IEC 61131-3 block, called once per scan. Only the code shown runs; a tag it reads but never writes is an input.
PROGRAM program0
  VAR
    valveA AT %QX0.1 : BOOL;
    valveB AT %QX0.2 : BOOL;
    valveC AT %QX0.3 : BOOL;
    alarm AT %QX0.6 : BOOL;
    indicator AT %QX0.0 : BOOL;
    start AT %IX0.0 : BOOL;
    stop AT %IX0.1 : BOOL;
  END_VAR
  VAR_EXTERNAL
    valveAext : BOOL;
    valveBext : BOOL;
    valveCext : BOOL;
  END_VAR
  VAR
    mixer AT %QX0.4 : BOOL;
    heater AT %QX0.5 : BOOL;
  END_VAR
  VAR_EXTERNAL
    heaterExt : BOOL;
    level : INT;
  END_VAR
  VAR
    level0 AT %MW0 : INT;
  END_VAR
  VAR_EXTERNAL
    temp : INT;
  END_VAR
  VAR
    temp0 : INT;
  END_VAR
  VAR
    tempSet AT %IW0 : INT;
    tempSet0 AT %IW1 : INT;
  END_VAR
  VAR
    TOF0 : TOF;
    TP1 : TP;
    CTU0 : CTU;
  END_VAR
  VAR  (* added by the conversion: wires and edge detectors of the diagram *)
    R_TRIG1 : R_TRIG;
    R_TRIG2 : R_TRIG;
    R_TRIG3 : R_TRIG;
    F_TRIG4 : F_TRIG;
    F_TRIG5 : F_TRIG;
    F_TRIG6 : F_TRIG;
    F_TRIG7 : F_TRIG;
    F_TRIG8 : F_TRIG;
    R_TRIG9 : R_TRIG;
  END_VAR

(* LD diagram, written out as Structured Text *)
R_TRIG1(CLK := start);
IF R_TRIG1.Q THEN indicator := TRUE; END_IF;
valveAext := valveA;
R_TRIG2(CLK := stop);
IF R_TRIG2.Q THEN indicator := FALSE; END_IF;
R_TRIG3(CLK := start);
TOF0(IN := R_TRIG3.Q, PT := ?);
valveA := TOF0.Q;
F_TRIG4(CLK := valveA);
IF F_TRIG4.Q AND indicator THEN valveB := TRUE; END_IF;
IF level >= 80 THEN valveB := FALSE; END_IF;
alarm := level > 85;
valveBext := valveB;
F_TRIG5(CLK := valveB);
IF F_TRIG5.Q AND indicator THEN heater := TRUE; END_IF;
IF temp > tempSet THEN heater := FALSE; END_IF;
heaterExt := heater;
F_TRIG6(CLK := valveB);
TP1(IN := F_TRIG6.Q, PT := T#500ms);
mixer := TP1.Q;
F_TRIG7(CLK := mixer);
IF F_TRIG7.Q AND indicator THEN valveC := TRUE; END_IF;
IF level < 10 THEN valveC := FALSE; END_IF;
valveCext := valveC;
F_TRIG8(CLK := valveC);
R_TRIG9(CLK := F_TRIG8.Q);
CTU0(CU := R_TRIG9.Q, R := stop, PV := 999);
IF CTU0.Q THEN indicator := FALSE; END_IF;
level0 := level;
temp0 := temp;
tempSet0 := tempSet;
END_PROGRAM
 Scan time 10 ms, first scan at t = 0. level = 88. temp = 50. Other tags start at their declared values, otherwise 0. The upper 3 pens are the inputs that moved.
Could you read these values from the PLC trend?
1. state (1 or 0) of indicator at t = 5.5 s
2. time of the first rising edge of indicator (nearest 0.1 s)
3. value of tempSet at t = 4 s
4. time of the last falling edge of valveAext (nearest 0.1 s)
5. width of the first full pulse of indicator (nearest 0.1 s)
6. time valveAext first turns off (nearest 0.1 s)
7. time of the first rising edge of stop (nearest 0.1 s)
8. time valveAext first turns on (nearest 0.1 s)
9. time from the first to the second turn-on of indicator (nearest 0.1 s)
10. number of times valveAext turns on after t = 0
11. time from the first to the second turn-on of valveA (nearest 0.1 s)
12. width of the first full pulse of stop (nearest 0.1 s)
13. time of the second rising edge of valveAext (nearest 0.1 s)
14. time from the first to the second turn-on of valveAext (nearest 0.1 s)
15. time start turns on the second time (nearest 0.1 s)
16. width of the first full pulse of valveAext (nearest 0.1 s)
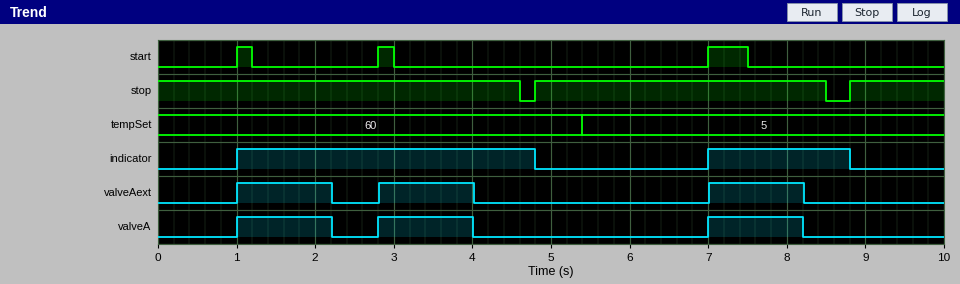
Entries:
0
1.0 s
60
8.2 s
3.8 s
2.2 s
4.8 s
1.0 s
6.0 s
3
1.8 s
3.7 s
2.8 s
1.8 s
2.8 s
1.2 s
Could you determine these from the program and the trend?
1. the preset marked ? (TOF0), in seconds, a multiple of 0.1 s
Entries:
1.2 s
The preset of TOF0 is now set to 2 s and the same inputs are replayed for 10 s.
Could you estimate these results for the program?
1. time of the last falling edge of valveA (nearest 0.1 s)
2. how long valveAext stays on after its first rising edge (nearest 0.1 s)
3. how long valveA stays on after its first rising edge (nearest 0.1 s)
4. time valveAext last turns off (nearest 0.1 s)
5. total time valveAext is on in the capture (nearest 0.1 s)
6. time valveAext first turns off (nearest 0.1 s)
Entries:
9.0 s
3.8 s
3.8 s
9.0 s
5.8 s
4.8 s
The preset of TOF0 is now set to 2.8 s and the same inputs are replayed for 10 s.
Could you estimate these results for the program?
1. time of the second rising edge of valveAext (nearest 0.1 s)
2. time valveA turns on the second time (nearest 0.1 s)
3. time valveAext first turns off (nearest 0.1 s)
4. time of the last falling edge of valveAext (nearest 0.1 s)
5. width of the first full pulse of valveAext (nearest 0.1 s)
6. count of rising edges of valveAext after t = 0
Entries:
7.0 s
7.0 s
5.6 s
9.8 s
4.6 s
2
